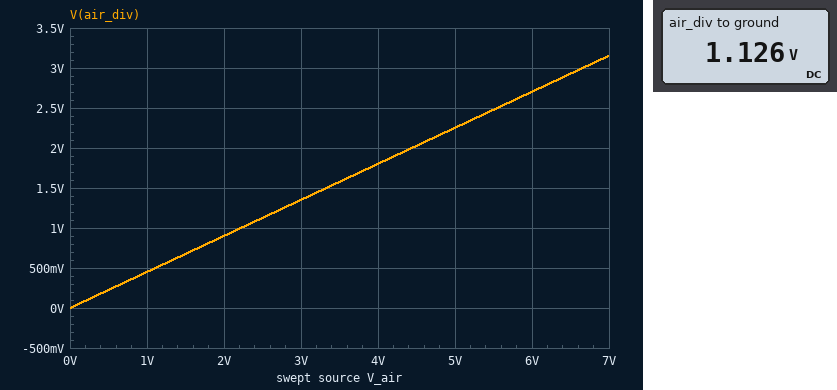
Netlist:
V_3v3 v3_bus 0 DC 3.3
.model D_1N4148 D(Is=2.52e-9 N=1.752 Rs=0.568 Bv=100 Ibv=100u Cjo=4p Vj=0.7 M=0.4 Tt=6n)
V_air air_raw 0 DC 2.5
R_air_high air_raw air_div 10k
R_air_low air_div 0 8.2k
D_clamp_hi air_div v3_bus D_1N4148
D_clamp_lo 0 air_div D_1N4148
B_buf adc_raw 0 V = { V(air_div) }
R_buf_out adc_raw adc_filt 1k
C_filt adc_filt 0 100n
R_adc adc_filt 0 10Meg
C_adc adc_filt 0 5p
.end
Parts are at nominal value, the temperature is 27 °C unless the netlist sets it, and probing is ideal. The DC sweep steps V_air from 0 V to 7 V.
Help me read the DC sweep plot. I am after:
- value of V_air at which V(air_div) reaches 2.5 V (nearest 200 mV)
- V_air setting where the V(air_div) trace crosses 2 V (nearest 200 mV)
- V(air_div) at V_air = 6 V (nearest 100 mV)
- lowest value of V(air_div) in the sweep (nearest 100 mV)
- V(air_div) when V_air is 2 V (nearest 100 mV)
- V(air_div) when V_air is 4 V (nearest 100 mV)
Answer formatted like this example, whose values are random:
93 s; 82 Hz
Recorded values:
5.6 V; 4.4 V; 2.7 V; 0 V; 900 mV; 1.8 V
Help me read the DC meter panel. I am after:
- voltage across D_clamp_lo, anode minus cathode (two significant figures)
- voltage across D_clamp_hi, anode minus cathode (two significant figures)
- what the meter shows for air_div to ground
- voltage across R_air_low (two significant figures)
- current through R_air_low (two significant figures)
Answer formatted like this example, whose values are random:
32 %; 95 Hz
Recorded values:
-1.1 V; -2.2 V; 1.126 V; 1.1 V; 140 µA
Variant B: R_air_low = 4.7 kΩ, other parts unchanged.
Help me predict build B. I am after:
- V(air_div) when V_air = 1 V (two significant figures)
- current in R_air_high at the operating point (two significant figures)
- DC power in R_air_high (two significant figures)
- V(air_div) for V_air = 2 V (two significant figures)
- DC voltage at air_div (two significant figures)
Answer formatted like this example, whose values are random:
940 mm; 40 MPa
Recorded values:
320 mV; 170 µA; 290 µW; 640 mV; 800 mV
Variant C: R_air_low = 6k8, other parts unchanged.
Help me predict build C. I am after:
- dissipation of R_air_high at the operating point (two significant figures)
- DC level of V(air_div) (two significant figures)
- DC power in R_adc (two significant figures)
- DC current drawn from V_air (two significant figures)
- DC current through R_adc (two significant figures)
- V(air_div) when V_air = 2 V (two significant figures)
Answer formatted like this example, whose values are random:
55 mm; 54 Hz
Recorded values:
220 µW; 1.0 V; 100 nW; 150 µA; 100 nA; 810 mV
